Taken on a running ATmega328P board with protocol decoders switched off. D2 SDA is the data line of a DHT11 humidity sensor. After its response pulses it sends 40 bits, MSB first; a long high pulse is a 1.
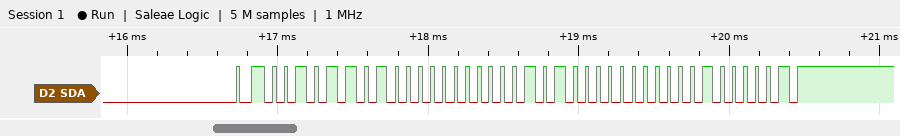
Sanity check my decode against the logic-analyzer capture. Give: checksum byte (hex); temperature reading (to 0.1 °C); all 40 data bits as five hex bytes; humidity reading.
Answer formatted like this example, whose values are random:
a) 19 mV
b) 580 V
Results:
a) 0x41
b) 20.0 °C
c) 2D 00 14 00 41
d) 45 %
